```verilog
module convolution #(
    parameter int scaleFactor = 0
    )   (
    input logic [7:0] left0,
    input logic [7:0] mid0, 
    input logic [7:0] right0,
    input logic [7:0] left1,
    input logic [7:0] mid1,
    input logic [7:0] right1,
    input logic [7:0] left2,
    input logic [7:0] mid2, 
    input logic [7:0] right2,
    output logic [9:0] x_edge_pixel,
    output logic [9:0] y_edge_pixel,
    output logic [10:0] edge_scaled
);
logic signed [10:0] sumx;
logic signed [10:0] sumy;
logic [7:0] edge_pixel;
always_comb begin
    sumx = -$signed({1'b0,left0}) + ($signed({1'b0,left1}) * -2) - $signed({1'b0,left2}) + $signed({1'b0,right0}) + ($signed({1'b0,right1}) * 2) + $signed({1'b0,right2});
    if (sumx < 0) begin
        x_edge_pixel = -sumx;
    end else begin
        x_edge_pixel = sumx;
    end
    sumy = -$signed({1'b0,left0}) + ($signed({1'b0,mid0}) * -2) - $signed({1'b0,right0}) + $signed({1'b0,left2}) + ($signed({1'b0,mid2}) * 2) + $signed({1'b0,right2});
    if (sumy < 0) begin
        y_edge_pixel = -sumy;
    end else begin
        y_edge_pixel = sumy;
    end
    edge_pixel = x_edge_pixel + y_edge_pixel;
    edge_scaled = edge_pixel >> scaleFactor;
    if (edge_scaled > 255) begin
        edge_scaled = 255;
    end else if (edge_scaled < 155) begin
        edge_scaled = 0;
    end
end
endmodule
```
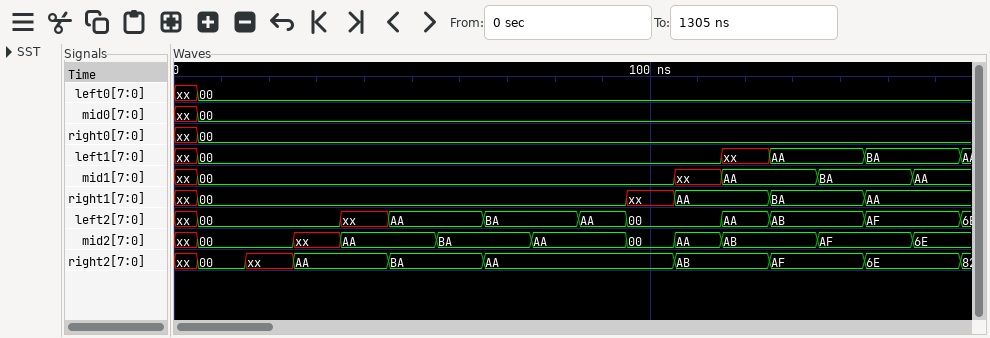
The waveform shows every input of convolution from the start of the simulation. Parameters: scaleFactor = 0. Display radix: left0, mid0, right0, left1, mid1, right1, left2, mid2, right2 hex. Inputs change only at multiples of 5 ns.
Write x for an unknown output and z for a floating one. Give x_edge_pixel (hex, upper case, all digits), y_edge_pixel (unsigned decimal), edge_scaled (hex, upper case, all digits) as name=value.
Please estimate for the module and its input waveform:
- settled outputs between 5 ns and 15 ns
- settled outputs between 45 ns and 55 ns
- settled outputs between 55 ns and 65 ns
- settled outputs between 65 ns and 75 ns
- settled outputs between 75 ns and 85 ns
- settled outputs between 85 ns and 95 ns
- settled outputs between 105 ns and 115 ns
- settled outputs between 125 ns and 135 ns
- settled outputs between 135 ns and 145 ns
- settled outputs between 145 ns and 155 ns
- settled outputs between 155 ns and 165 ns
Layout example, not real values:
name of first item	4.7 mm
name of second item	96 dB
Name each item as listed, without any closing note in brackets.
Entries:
settled outputs between 5 ns and 15 ns	x_edge_pixel=000, y_edge_pixel=0, edge_scaled=000
settled outputs between 45 ns and 55 ns	x_edge_pixel=010, y_edge_pixel=696, edge_scaled=0C8
settled outputs between 55 ns and 65 ns	x_edge_pixel=010, y_edge_pixel=728, edge_scaled=0E8
settled outputs between 65 ns and 75 ns	x_edge_pixel=010, y_edge_pixel=728, edge_scaled=0E8
settled outputs between 75 ns and 85 ns	x_edge_pixel=010, y_edge_pixel=696, edge_scaled=0C8
settled outputs between 85 ns and 95 ns	x_edge_pixel=000, y_edge_pixel=680, edge_scaled=0A8
settled outputs between 105 ns and 115 ns	x_edge_pixel=1FF, y_edge_pixel=511, edge_scaled=0FE
settled outputs between 125 ns and 135 ns	x_edge_pixel=024, y_edge_pixel=688, edge_scaled=0D4
settled outputs between 135 ns and 145 ns	x_edge_pixel=024, y_edge_pixel=696, edge_scaled=0DC
settled outputs between 145 ns and 155 ns	x_edge_pixel=061, y_edge_pixel=635, edge_scaled=0DC
settled outputs between 155 ns and 165 ns	x_edge_pixel=061, y_edge_pixel=505, edge_scaled=000
